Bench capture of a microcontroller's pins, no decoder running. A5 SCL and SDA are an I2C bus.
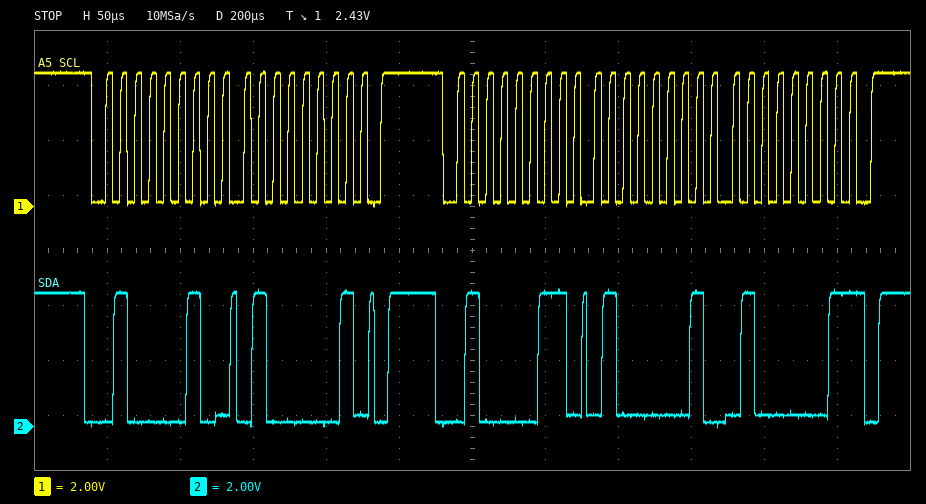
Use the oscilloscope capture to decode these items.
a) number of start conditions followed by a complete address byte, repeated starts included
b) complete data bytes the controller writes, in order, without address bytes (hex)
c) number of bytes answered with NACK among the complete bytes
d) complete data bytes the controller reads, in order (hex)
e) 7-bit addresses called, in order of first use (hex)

2
41
1
41 41
0x21
